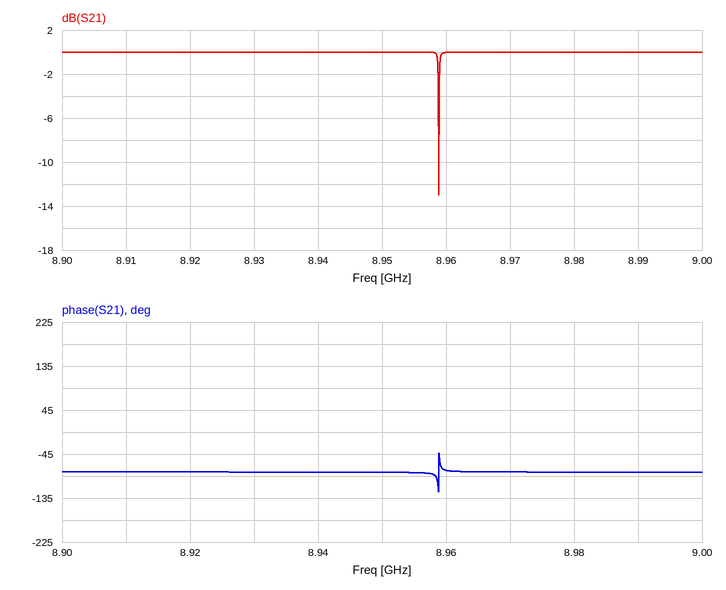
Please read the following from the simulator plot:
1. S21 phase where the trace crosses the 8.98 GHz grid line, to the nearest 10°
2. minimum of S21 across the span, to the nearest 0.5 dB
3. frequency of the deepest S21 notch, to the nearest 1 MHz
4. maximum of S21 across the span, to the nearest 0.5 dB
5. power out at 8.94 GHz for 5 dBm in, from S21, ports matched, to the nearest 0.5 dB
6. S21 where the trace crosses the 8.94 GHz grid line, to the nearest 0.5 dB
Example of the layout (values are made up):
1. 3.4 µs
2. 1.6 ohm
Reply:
1. -80°
2. -13.0 dB
3. 8.959 GHz
4. 0.0 dB
5. 5.0 dBm
6. 0.0 dB
